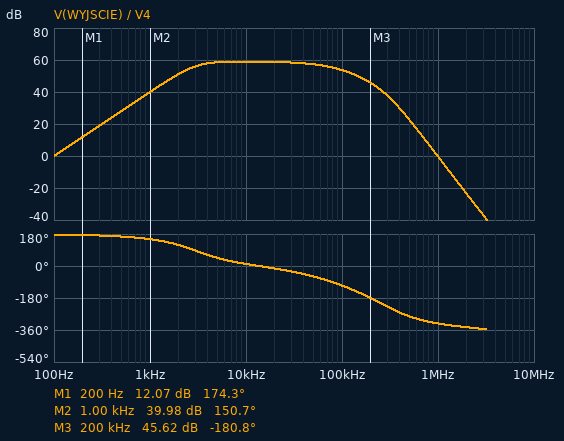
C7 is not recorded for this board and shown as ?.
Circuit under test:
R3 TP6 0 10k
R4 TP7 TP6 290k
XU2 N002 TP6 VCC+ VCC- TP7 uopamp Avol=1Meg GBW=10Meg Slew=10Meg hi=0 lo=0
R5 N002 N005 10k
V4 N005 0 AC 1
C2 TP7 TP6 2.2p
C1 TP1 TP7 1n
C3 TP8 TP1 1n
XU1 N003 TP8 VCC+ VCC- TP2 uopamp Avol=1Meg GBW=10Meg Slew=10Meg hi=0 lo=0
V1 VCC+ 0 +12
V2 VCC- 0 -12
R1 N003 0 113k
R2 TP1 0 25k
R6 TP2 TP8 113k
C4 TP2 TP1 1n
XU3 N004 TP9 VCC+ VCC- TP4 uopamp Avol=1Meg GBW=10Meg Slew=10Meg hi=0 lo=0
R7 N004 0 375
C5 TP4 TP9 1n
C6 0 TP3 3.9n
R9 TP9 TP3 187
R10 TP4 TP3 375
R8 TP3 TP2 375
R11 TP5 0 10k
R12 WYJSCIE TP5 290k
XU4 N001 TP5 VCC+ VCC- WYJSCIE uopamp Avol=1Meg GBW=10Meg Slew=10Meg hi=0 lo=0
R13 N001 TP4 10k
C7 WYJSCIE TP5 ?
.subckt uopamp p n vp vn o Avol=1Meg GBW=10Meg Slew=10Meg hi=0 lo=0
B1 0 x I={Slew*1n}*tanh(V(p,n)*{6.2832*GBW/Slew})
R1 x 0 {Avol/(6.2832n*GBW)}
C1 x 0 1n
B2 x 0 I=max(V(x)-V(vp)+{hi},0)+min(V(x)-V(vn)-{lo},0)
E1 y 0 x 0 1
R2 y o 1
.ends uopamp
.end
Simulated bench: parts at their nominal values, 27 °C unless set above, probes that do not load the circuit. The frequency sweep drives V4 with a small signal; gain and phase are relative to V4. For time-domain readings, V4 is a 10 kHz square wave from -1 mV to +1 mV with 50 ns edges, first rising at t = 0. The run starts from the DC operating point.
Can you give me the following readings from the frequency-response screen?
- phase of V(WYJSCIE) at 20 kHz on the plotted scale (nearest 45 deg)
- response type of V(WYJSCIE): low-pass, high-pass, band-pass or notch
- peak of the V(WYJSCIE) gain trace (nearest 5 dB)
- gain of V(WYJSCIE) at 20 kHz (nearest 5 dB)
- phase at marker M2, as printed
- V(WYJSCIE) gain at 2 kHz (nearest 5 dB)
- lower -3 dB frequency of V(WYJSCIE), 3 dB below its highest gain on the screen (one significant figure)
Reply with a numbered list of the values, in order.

1. 0 deg
2. band-pass
3. 60 dB
4. 60 dB
5. 150.7 deg
6. 50 dB
7. 3 kHz
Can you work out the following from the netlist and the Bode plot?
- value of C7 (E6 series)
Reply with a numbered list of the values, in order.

1. 4.7 pF
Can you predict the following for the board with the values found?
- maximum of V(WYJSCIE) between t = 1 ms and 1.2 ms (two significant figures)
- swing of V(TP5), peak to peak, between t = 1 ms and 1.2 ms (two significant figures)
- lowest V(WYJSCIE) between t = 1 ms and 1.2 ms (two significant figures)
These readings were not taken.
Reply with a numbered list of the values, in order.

1. 1.3 V
2. 87 mV
3. -1.3 V
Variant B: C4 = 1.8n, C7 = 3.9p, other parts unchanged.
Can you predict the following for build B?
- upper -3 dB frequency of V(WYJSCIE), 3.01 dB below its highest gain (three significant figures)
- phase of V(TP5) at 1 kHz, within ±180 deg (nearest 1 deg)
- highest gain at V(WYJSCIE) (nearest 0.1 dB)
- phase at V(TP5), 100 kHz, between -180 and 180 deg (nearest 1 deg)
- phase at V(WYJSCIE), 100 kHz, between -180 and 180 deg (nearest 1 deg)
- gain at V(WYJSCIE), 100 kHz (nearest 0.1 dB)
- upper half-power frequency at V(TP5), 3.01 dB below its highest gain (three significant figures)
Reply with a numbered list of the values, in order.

1. 74.7 kHz
2. 142 deg
3. 54.0 dB
4. -73 deg
5. -107 deg
6. 49.2 dB
7. 99.2 kHz
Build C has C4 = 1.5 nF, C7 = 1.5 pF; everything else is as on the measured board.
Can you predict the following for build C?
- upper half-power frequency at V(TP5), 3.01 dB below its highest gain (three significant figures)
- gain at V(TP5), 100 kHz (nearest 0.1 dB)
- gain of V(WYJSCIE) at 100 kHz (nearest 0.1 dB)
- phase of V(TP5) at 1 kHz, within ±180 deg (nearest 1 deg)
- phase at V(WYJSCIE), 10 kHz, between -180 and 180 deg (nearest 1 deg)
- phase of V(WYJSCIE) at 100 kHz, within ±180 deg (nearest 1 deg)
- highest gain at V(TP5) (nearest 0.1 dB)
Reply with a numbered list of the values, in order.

1. 107 kHz
2. 23.4 dB
3. 52.6 dB
4. 146 deg
5. 9 deg
6. -92 deg
7. 26.0 dB
